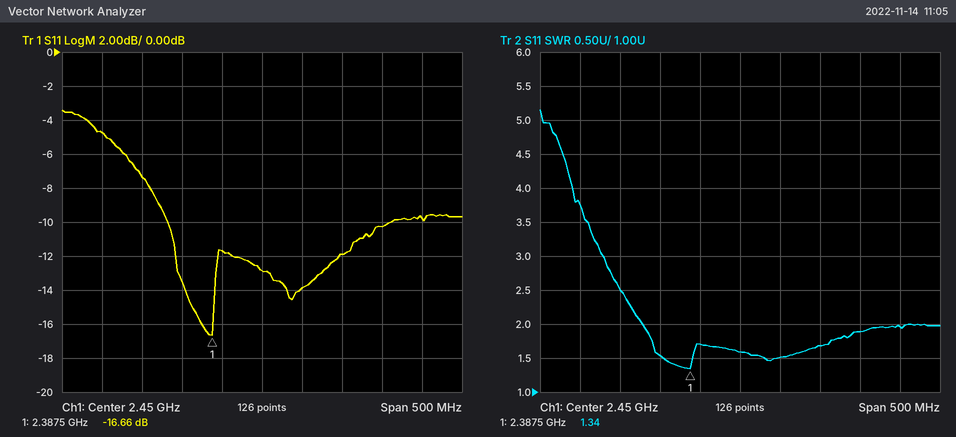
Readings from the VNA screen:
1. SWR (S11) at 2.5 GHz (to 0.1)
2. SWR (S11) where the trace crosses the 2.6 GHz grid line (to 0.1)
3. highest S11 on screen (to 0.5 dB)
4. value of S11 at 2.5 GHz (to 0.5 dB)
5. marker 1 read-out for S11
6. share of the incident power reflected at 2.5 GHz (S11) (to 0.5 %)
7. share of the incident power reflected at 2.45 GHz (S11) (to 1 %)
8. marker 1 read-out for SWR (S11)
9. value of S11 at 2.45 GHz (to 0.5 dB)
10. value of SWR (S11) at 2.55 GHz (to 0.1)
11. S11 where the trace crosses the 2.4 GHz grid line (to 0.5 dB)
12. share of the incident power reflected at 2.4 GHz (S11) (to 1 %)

1.5
1.9
-3.5 dB
-14.0 dB
-16.66 dB
4.0 %
5 %
1.34
-13.0 dB
1.7
-11.5 dB
7 %
